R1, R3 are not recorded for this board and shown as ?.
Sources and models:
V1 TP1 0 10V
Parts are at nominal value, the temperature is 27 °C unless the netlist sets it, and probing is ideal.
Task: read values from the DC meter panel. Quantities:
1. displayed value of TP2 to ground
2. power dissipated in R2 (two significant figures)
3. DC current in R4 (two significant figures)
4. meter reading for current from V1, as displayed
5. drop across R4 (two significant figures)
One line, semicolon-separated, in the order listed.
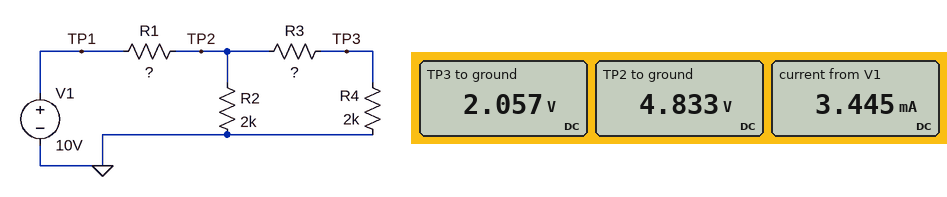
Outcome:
4.833 V; 12 mW; 1.0 mA; 3.445 mA; 2.1 V
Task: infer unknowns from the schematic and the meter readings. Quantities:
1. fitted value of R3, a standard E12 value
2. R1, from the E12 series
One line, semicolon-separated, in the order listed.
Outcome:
2.7 kΩ; 1.5 kΩ
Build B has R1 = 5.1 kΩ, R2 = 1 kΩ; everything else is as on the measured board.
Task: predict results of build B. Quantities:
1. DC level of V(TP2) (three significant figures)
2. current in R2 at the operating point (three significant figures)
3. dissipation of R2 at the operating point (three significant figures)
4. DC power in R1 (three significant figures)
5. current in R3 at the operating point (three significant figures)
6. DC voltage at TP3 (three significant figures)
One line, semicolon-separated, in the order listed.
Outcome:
1.39 V; 1.39 mA; 1.94 mW; 14.5 mW; 296 µA; 592 mV
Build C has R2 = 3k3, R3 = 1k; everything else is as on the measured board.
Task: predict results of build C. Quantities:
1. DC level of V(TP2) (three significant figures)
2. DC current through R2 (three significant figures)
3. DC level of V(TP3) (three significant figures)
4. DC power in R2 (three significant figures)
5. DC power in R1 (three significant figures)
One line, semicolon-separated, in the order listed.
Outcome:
5.12 V; 1.55 mA; 3.41 V; 7.93 mW; 15.9 mW
